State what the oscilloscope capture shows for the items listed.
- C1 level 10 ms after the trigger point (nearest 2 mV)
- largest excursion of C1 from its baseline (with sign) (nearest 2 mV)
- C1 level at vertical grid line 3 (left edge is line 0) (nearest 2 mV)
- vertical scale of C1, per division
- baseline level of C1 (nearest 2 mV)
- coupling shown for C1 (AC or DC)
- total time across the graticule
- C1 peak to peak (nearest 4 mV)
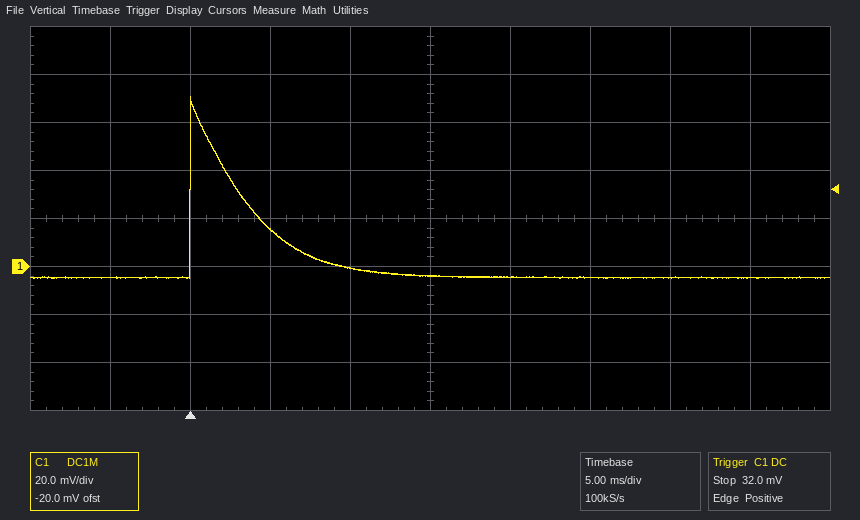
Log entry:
0 mV
+76 mV
16 mV
20 mV
-4 mV
DC
50 ms
76 mV
